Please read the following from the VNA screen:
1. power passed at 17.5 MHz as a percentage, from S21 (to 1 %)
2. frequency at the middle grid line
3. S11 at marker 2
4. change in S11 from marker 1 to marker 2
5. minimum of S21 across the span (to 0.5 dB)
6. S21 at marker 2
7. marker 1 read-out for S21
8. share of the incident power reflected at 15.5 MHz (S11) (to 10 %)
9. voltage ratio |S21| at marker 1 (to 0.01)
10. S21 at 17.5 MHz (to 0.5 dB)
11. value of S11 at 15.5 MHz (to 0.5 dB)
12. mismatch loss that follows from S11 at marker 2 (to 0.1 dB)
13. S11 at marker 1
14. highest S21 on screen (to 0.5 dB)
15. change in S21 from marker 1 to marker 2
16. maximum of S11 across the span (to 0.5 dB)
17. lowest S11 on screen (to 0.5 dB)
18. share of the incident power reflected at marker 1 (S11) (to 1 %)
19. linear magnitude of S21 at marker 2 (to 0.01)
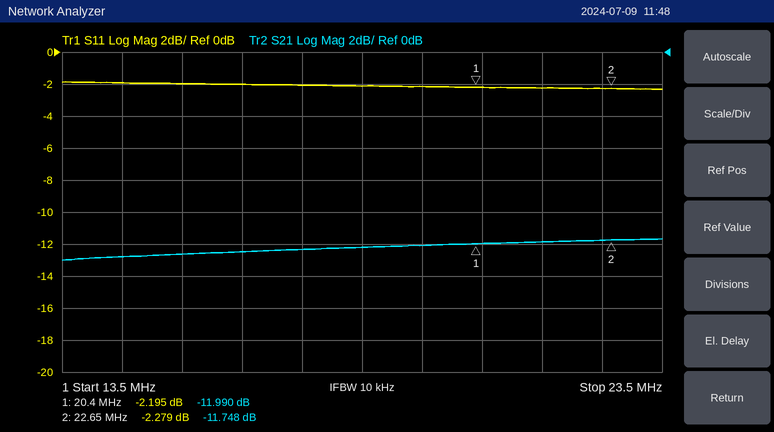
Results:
6 %
18.5 MHz
-2.279 dB
-0.084 dB
-13.0 dB
-11.748 dB
-11.990 dB
60 %
0.25
-12.5 dB
-2.0 dB
3.9 dB
-2.195 dB
-11.5 dB
0.242 dB
-2.0 dB
-2.5 dB
60 %
0.26
